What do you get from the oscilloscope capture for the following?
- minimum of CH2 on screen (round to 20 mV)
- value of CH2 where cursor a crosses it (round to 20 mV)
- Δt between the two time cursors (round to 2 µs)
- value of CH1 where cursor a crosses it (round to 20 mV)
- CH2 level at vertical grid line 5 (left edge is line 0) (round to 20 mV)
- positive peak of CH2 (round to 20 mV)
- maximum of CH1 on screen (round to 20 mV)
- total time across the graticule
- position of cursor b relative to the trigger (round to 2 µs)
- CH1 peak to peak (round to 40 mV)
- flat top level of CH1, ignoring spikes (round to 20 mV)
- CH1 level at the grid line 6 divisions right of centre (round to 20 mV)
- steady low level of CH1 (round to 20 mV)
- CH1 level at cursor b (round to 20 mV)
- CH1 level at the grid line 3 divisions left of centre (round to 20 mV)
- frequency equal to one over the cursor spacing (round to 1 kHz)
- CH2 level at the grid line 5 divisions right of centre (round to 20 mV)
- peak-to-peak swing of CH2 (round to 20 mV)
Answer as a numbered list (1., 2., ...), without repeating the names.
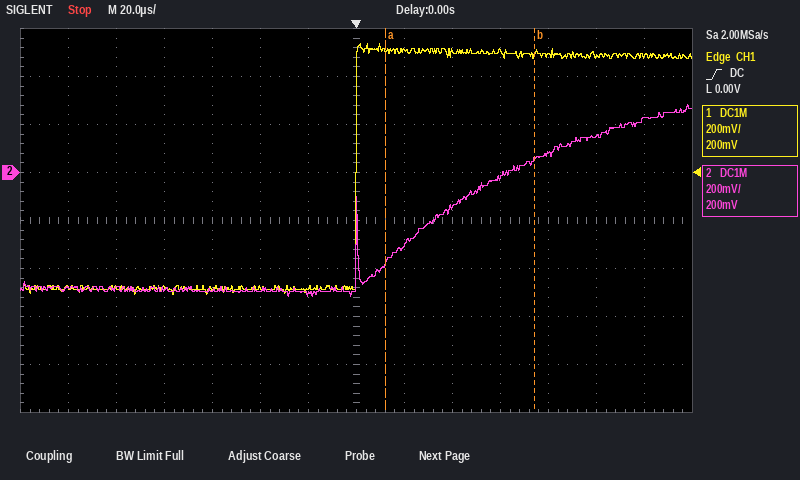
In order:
1. -520 mV
2. -380 mV
3. 62 µs
4. 500 mV
5. -500 mV
6. 280 mV
7. 540 mV
8. 280 µs
9. +74 µs
10. 1.04 V
11. 500 mV
12. 480 mV
13. -480 mV
14. 500 mV
15. -480 mV
16. 16 kHz
17. 160 mV
18. 800 mV
